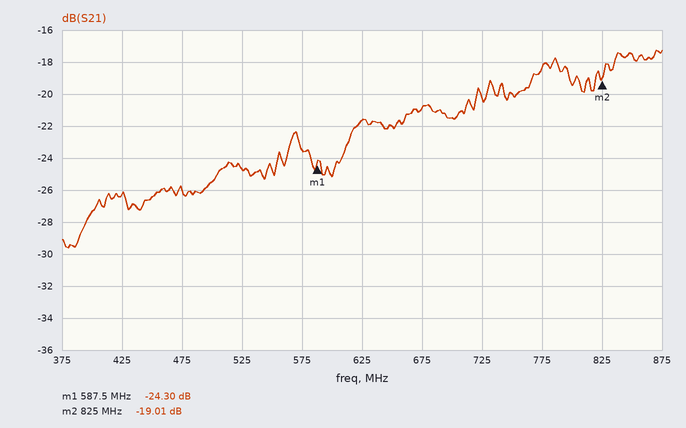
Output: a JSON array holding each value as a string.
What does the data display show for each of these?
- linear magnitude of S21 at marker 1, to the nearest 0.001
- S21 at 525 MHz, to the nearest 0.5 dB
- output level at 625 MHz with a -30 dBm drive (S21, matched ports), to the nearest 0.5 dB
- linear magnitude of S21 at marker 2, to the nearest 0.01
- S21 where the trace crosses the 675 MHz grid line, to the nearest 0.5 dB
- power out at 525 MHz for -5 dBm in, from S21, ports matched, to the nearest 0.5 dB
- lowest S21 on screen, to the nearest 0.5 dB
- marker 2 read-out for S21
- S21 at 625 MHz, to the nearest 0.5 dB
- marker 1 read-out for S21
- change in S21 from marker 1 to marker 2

["0.061", "-24.5 dB", "-51.5 dBm", "0.11", "-21.0 dB", "-29.5 dBm", "-29.5 dB", "-19.01 dB", "-21.5 dB", "-24.30 dB", "5.29 dB"]
